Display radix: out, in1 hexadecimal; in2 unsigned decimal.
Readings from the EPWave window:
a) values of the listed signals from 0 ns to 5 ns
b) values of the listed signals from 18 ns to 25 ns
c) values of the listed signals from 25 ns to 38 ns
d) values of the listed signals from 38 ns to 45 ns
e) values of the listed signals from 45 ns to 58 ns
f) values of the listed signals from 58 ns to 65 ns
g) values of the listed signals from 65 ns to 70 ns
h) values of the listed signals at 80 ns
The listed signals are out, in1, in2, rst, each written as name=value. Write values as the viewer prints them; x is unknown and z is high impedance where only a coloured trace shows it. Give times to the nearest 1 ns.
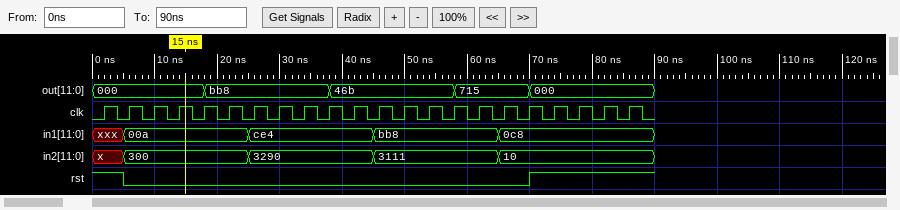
out=000, in1=xxx, in2=x, rst=1
out=bb8, in1=00a, in2=300, rst=0
out=bb8, in1=ce4, in2=3290, rst=0
out=46b, in1=ce4, in2=3290, rst=0
out=46b, in1=bb8, in2=3111, rst=0
out=715, in1=bb8, in2=3111, rst=0
out=715, in1=0c8, in2=10, rst=0
out=000, in1=0c8, in2=10, rst=1
